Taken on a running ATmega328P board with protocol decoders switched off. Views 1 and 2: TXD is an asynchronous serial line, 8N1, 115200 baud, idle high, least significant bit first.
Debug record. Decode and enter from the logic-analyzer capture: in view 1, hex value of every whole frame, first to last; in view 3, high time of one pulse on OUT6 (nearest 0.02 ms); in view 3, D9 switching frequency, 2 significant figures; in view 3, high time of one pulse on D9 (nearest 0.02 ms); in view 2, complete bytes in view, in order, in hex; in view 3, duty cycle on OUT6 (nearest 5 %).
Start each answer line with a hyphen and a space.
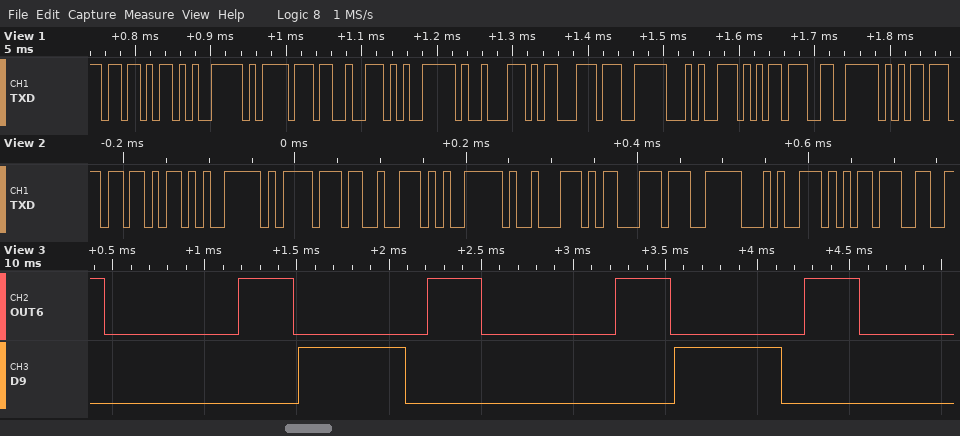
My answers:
- 5B E5 BD 93 E5 89 8D E7 94 B5 E6 B5
- 0.30 ms
- 490 Hz
- 0.58 ms
- 5B E5 BD 93 E5 89 8D E7 94 B5
- 30 %
